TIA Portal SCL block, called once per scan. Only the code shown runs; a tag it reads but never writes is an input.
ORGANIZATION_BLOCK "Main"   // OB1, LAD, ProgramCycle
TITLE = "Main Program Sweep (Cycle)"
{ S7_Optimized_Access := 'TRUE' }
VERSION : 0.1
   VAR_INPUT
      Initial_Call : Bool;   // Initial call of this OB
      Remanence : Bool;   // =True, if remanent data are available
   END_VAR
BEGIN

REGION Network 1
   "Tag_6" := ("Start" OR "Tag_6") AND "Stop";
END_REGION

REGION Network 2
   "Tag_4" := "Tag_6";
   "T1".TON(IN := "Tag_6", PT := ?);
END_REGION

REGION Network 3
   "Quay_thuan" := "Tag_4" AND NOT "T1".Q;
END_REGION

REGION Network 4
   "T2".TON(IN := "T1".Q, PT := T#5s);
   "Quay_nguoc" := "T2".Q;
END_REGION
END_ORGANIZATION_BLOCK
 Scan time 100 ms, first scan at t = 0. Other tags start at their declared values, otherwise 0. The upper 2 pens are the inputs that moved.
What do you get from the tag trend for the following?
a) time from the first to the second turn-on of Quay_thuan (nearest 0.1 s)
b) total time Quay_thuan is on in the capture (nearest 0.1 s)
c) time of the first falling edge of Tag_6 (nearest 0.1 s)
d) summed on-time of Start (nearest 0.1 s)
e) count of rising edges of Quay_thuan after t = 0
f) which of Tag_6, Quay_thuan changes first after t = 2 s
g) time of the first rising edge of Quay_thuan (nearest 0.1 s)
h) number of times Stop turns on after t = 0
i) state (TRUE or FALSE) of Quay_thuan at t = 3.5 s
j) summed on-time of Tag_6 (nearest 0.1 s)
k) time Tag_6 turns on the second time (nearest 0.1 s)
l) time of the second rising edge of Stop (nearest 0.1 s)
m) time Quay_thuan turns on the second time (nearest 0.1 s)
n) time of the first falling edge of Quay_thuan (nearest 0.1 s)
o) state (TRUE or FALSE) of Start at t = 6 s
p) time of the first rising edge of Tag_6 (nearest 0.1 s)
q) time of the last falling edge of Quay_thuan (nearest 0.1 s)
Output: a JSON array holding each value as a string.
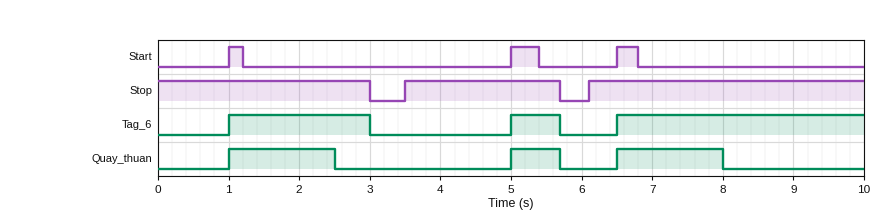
["4.0 s", "3.7 s", "3.0 s", "0.9 s", "3", "Quay_thuan", "1.0 s", "2", "FALSE", "6.2 s", "5.0 s", "6.1 s", "5.0 s", "2.5 s", "FALSE", "1.0 s", "8.0 s"]
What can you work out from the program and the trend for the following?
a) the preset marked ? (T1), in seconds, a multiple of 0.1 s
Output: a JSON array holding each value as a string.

["1.5 s"]
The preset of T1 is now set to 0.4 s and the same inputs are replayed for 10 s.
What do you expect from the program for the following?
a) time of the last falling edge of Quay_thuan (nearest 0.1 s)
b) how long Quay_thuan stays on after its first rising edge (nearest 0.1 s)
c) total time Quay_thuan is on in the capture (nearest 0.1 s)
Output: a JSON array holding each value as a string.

["6.9 s", "0.4 s", "1.2 s"]
